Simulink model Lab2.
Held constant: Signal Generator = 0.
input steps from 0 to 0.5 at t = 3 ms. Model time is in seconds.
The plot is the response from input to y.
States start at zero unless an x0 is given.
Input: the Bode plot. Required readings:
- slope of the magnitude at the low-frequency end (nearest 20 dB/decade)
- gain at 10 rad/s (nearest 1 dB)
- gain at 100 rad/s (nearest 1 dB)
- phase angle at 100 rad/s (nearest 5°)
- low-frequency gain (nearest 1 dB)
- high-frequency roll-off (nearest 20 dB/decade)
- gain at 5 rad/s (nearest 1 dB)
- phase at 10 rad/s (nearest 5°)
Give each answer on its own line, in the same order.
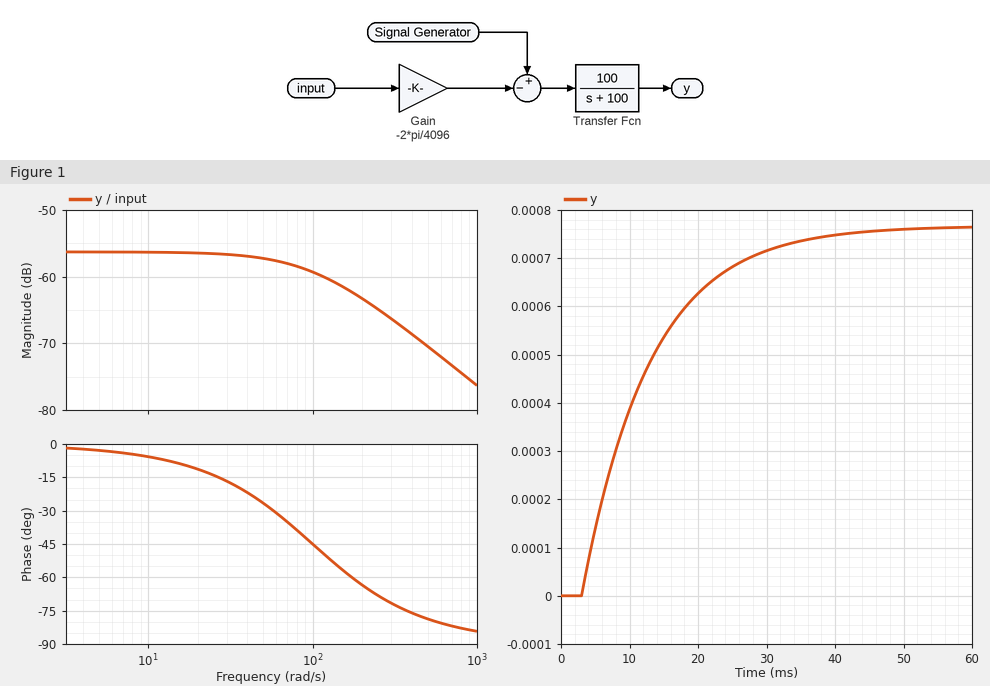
0 dB/decade
-56 dB
-59 dB
-45°
-56 dB
-20 dB/decade
-56 dB
-5°
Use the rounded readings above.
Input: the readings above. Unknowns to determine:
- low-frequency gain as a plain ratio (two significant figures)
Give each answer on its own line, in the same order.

0.0016
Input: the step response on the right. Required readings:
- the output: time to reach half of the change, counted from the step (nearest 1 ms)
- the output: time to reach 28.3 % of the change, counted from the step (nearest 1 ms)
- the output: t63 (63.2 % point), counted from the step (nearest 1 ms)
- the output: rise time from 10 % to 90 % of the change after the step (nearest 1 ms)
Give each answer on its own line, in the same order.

7 ms
3 ms
10 ms
22 ms
